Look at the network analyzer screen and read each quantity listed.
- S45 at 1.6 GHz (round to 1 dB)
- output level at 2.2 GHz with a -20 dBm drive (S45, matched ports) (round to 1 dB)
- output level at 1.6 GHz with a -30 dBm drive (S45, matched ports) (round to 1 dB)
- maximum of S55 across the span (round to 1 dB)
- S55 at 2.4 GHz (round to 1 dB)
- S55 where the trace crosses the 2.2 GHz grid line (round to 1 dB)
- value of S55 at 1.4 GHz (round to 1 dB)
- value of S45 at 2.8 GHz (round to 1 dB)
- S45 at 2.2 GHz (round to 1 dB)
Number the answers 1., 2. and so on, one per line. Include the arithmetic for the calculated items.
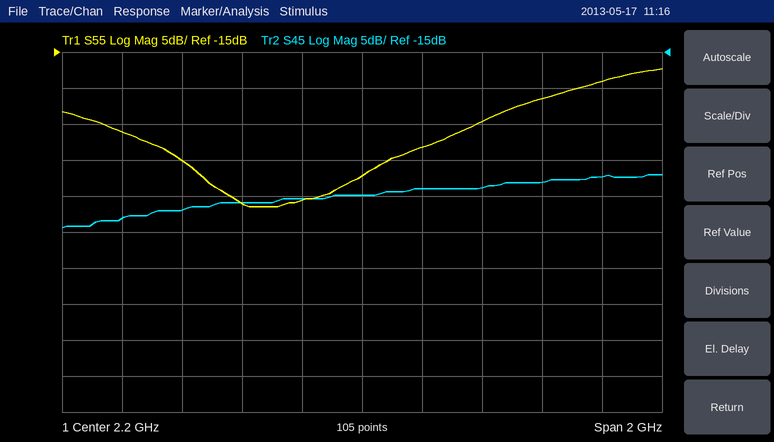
1. -37 dB
2. -20 dBm + (-35 dB) = -55 dBm
3. -30 dBm + (-37 dB) = -67 dBm
4. -17 dB
5. -28 dB
6. -32 dB
7. -26 dB
8. -33 dB
9. -35 dB
